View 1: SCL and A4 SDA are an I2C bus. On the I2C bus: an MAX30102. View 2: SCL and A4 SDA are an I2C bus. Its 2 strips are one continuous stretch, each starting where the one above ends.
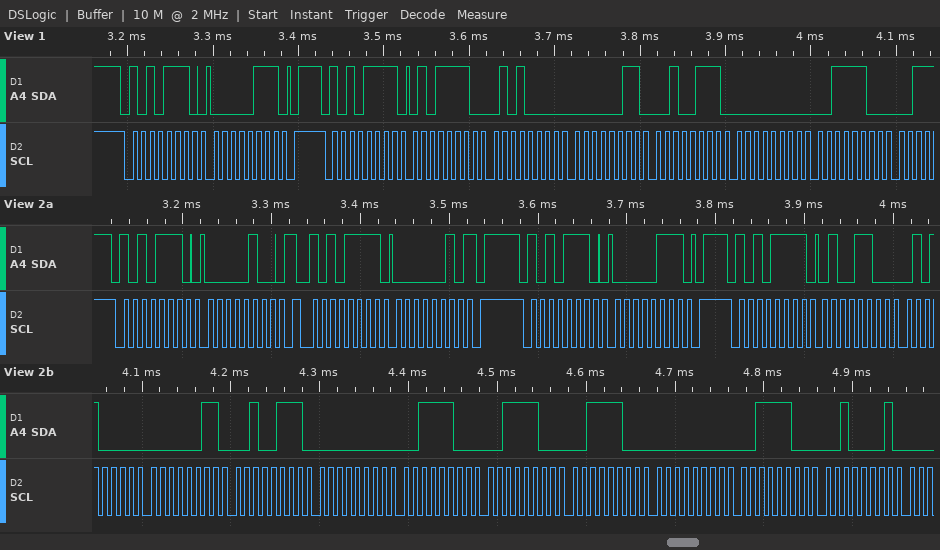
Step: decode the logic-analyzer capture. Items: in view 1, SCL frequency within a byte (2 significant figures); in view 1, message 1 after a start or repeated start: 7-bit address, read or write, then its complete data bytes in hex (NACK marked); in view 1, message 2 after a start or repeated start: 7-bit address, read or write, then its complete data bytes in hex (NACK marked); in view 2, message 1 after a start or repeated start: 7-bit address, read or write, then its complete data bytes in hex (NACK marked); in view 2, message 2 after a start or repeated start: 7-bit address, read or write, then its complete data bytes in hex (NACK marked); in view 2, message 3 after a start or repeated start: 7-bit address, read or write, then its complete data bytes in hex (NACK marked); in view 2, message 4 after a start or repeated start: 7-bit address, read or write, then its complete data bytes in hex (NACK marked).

100 kHz
0x57 write: 07
0x57 read: 5E 50 03 27 00 3C
0x57 write: 04
0x57 read: 02 NACK
0x57 write: 07
0x57 read: 4C 50 03 27 00 3C 3C 3C 00 3C 21
